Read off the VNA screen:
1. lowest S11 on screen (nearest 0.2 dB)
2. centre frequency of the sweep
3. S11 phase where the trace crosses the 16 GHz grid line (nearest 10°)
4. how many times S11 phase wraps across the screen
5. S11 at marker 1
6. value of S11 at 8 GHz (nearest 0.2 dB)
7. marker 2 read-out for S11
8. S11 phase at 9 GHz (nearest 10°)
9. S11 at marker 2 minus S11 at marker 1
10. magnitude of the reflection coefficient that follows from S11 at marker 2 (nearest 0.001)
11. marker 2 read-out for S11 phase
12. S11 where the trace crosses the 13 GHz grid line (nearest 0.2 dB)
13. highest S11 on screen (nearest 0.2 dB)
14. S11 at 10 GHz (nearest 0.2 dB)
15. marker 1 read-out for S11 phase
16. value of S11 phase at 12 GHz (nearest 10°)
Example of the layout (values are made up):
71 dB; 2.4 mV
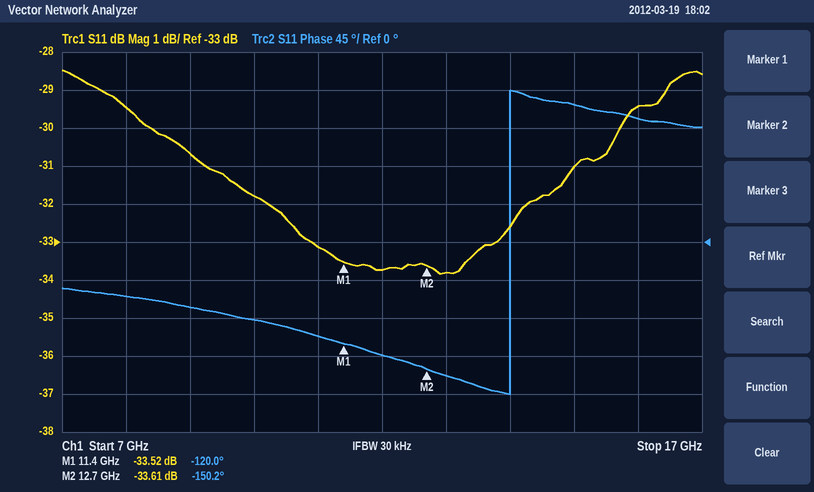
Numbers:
-33.8 dB; 12 GHz; 150°; 1; -33.52 dB; -29.4 dB; -33.61 dB; -80°; -0.09 dB; 0.021; -150.2°; -33.8 dB; -28.4 dB; -31.8 dB; -120.0°; -130°
